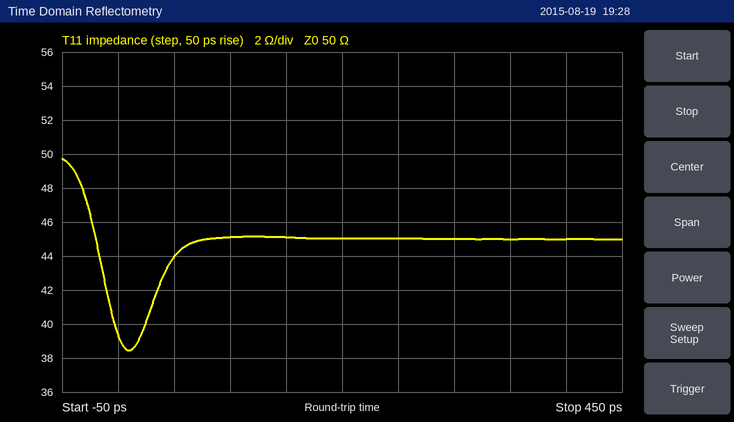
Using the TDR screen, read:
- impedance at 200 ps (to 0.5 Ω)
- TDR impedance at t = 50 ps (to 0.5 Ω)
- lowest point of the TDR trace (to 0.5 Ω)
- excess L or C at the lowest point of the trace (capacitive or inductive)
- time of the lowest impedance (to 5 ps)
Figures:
45.0 Ω
44.0 Ω
38.5 Ω
capacitive
10 ps
